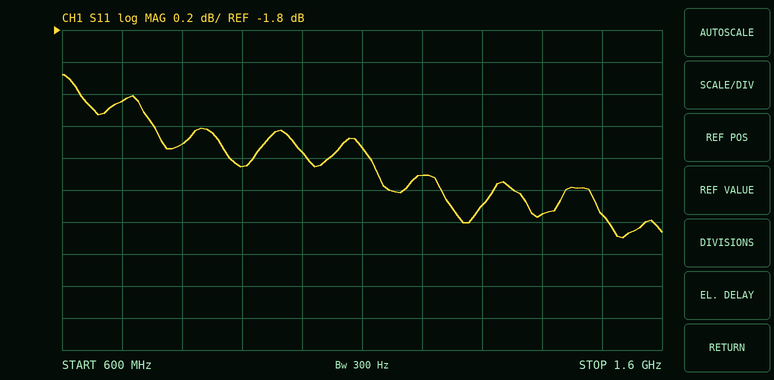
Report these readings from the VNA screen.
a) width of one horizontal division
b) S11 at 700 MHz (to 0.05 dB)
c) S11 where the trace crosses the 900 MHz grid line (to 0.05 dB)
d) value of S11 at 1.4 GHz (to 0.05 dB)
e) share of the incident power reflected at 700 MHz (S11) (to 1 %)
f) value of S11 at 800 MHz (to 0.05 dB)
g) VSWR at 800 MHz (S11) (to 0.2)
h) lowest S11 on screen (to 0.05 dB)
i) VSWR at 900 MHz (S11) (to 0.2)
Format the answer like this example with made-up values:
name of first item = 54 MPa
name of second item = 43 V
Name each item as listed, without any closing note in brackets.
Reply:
width of one horizontal division = 100 MHz
S11 at 700 MHz = -2.25 dB
S11 where the trace crosses the 900 MHz grid line = -2.65 dB
value of S11 at 1.4 GHz = -2.95 dB
share of the incident power reflected at 700 MHz (S11) = 60 %
value of S11 at 800 MHz = -2.50 dB
VSWR at 800 MHz (S11) = 7.0
lowest S11 on screen = -3.10 dB
VSWR at 900 MHz (S11) = 6.6
